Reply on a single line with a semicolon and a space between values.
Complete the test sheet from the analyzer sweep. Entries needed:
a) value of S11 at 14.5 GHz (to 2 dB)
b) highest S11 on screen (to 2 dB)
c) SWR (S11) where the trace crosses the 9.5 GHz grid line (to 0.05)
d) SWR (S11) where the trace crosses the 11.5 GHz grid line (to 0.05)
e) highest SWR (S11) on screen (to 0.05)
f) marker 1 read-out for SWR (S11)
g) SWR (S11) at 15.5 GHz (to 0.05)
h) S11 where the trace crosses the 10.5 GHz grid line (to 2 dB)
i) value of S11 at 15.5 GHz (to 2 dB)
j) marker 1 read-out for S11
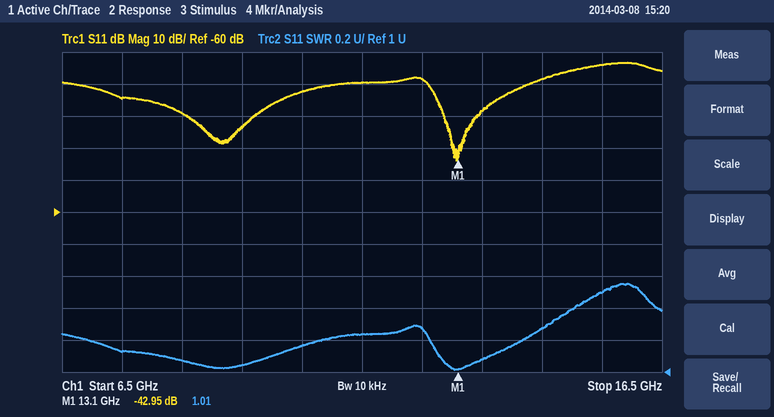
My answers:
-18 dB; -14 dB; 1.05; 1.25; 1.55; 1.01; 1.50; -22 dB; -14 dB; -42.95 dB
